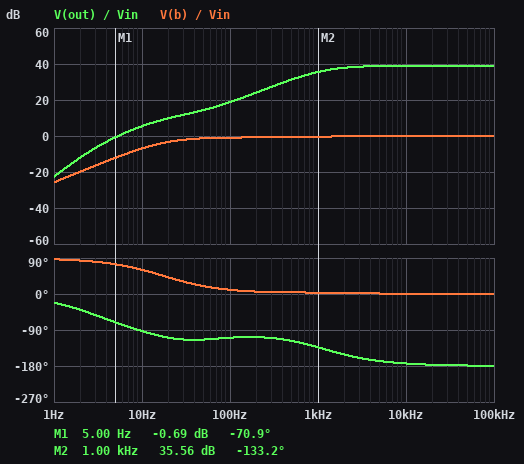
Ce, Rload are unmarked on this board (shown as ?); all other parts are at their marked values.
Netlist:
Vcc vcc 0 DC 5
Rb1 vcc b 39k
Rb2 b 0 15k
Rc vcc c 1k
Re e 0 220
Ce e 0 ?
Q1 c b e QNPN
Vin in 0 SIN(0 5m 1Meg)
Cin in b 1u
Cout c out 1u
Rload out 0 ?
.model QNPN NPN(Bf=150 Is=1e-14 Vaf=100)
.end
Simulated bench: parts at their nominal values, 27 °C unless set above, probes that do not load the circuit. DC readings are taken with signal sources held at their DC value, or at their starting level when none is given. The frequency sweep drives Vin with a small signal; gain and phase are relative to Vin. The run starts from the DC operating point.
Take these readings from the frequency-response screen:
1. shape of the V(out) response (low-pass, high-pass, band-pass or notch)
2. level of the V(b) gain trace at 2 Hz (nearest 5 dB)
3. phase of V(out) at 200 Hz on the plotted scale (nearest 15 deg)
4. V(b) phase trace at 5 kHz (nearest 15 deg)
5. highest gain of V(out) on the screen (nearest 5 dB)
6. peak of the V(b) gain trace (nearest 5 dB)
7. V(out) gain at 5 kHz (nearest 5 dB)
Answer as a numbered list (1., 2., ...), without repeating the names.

1. high-pass
2. -20 dB
3. -105 deg
4. 0 deg
5. 40 dB
6. 0 dB
7. 40 dB
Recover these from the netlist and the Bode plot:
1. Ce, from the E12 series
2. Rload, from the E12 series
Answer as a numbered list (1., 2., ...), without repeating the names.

1. 15 µF
2. 56 kΩ
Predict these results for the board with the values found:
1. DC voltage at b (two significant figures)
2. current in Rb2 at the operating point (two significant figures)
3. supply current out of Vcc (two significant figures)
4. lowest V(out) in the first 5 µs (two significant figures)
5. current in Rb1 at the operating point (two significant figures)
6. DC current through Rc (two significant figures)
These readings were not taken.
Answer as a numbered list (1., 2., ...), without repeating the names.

1. 1.2 V
2. 81 µA
3. 2.5 mA
4. -490 mV
5. 97 µA
6. 2.4 mA
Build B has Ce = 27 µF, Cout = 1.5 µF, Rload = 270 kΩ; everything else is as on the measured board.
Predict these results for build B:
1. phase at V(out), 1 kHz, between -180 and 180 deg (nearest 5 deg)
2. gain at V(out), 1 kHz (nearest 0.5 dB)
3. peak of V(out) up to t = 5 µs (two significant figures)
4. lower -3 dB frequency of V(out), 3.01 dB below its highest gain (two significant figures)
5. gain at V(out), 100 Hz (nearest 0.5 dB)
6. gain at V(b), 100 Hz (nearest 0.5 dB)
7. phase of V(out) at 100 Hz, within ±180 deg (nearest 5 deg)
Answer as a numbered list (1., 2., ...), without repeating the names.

1. -145 deg
2. 37.5 dB
3. 420 mV
4. 670 Hz
5. 23.0 dB
6. -1.5 dB
7. -105 deg
